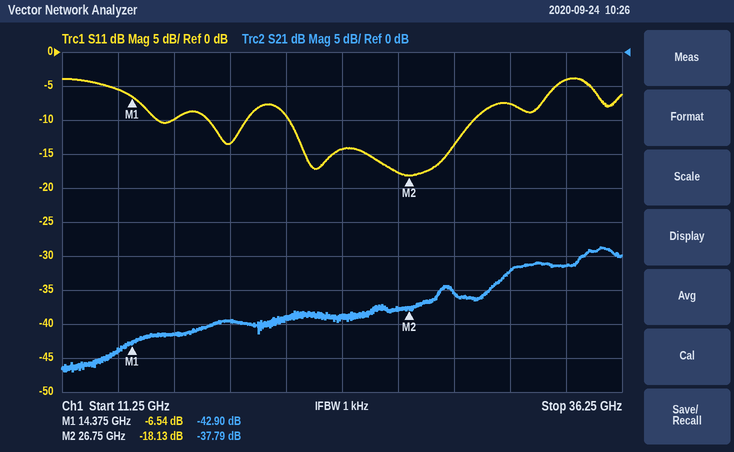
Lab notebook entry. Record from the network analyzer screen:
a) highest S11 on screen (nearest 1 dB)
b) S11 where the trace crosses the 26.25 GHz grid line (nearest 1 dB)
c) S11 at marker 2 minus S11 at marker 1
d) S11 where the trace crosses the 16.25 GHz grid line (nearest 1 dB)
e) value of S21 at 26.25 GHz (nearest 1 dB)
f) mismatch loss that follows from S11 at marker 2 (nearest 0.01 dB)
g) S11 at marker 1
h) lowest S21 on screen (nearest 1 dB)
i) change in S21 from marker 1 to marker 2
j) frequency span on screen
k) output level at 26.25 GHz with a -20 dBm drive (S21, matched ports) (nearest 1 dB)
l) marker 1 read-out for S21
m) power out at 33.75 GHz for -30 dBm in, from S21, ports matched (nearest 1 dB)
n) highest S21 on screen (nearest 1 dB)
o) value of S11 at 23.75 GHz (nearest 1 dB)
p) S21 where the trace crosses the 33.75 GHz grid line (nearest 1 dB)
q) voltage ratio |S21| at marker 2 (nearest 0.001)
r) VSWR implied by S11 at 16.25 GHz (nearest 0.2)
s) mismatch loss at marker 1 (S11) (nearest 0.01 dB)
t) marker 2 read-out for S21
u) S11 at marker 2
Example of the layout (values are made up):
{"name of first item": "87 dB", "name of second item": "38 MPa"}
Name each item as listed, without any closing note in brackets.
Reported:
{"highest S11 on screen": "-4 dB", "S11 where the trace crosses the 26.25 GHz grid line": "-18 dB", "S11 at marker 2 minus S11 at marker 1": "-11.59 dB", "S11 where the trace crosses the 16.25 GHz grid line": "-10 dB", "value of S21 at 26.25 GHz": "-38 dB", "mismatch loss that follows from S11 at marker 2": "0.07 dB", "S11 at marker 1": "-6.54 dB", "lowest S21 on screen": "-47 dB", "change in S21 from marker 1 to marker 2": "5.11 dB", "frequency span on screen": "25 GHz", "output level at 26.25 GHz with a -20 dBm drive (S21, matched ports)": "-58 dBm", "marker 1 read-out for S21": "-42.90 dB", "power out at 33.75 GHz for -30 dBm in, from S21, ports matched": "-61 dBm", "highest S21 on screen": "-29 dB", "value of S11 at 23.75 GHz": "-14 dB", "S21 where the trace crosses the 33.75 GHz grid line": "-31 dB", "voltage ratio |S21| at marker 2": "0.013", "VSWR implied by S11 at 16.25 GHz": "2.0", "mismatch loss at marker 1 (S11)": "1.09 dB", "marker 2 read-out for S21": "-37.79 dB", "S11 at marker 2": "-18.13 dB"}
